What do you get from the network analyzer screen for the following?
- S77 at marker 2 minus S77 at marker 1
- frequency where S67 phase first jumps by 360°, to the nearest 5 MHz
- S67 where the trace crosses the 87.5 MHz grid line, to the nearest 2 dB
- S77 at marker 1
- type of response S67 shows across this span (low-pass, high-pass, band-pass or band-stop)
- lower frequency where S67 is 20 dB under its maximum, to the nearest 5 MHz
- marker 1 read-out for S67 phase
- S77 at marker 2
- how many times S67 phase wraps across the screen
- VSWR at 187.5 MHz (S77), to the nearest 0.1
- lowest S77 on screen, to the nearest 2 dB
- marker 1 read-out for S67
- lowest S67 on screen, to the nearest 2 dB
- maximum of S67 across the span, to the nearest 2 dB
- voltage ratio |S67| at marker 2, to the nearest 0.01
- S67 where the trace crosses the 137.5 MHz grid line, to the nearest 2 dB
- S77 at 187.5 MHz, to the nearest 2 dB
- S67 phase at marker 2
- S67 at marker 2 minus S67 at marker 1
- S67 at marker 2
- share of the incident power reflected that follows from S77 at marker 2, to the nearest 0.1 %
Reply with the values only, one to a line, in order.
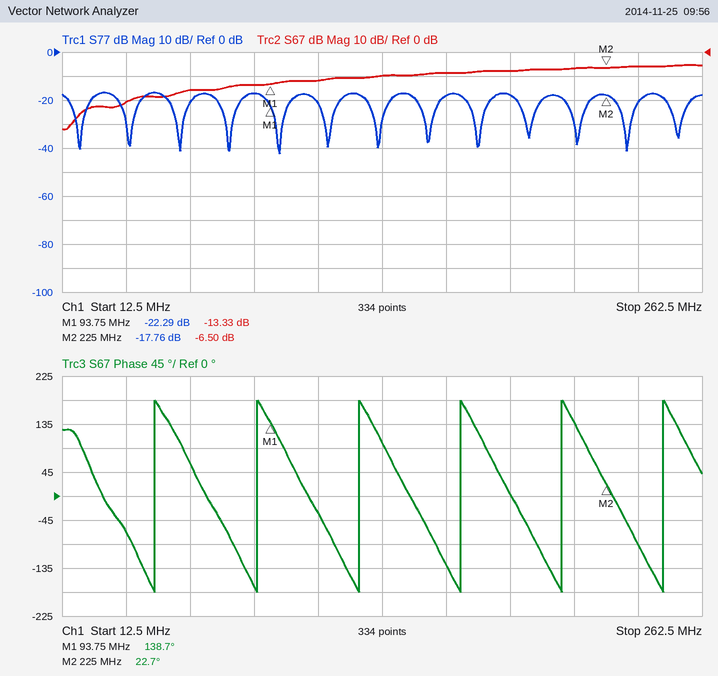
4.53 dB
50 MHz
-14 dB
-22.29 dB
high-pass
20 MHz
138.7°
-17.76 dB
6
1.3
-42 dB
-13.33 dB
-32 dB
-6 dB
0.47
-10 dB
-18 dB
22.7°
6.83 dB
-6.50 dB
1.7 %
